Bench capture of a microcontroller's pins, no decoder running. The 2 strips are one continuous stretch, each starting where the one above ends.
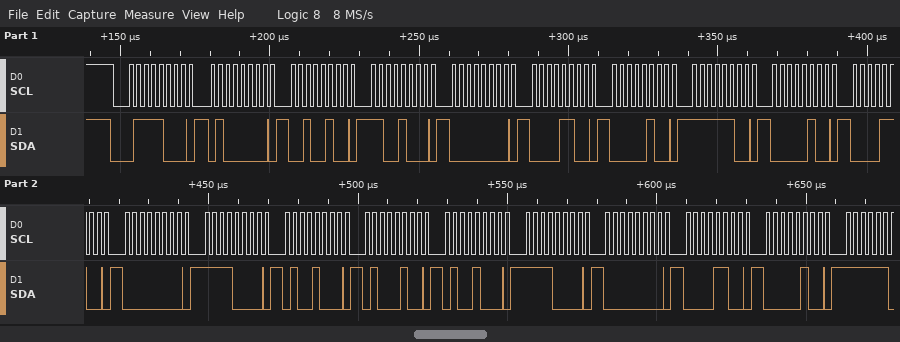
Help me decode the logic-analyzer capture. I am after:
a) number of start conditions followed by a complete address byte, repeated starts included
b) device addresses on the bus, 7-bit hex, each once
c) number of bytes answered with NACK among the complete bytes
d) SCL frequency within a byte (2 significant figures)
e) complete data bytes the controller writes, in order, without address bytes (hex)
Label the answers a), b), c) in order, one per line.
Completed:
a) 1
b) 0x3C
c) 0
d) 400 kHz
e) 40 24 C8 00 0C 04 FC 04 0C 00 F0 48 44 48 F0 00 0C 04
